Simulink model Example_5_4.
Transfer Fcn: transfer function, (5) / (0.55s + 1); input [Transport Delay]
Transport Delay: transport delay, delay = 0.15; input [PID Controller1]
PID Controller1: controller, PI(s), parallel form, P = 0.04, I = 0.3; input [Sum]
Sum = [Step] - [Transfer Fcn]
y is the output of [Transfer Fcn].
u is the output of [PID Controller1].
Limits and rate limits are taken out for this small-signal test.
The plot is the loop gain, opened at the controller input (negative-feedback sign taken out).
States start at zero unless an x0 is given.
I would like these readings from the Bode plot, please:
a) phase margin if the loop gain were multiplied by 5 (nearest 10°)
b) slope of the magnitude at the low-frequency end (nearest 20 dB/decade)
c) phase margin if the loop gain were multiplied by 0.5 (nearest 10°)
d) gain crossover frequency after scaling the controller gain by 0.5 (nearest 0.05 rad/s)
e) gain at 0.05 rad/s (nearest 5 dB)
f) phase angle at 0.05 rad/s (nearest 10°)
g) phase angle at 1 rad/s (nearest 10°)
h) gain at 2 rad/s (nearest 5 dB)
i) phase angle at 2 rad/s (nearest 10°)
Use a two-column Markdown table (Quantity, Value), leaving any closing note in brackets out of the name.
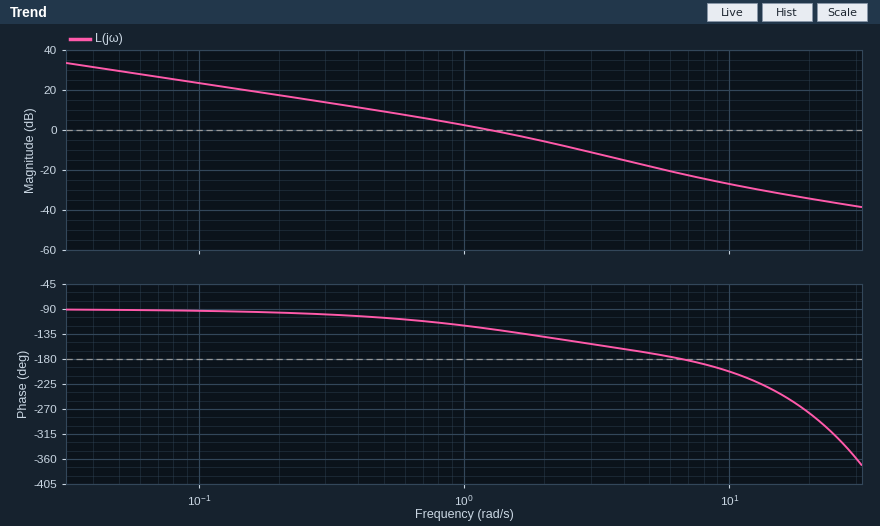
| Quantity | Value |
|---|---|
| phase margin if the loop gain were multiplied by 5 | 20° |
| slope of the magnitude at the low-frequency end | -20 dB/decade |
| phase margin if the loop gain were multiplied by 0.5 | 70° |
| gain crossover frequency after scaling the controller gain by 0.5 | 0.70 rad/s |
| gain at 0.05 rad/s | 30 dB |
| phase angle at 0.05 rad/s | -90° |
| phase angle at 1 rad/s | -120° |
| gain at 2 rad/s | -5 dB |
| phase angle at 2 rad/s | -140° |
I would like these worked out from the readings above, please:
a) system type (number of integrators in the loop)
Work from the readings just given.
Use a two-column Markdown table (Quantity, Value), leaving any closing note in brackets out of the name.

| Quantity | Value |
|---|---|
| system type | 1 |
